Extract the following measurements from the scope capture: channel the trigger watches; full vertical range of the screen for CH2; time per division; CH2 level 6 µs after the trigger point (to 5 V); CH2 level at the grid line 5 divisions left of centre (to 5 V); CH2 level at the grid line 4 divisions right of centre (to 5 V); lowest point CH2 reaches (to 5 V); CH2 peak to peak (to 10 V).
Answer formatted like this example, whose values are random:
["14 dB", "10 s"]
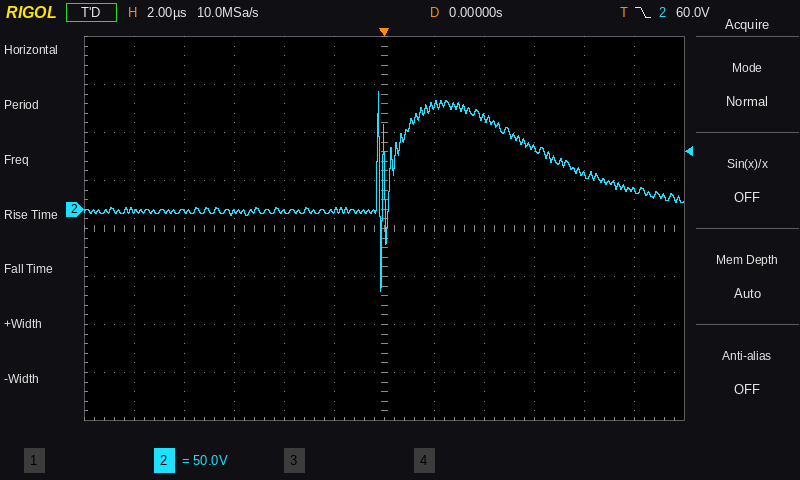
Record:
["CH2", "400 V", "2 µs", "65 V", "0 V", "35 V", "-85 V", "210 V"]
